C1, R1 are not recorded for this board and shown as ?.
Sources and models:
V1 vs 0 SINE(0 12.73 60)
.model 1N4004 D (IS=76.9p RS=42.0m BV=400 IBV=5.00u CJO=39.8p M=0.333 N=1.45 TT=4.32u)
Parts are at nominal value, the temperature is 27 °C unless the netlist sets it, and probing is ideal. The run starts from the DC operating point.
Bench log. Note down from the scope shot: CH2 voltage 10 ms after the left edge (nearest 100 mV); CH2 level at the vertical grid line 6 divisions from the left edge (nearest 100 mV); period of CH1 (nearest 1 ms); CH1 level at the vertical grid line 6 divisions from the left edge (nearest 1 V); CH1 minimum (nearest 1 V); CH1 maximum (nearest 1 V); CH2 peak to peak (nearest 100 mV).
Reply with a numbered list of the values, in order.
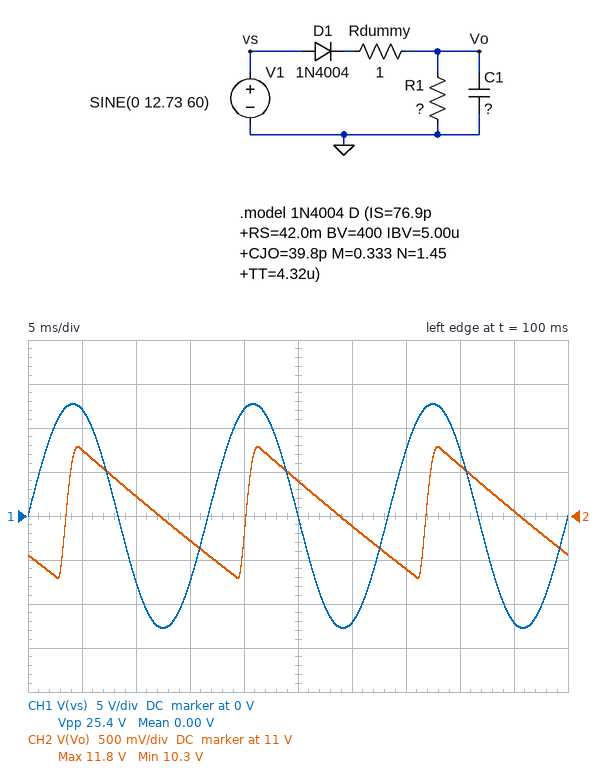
1. 11.2 V
2. 10.9 V
3. 17 ms
4. -12 V
5. -13 V
6. 13 V
7. 1.5 V
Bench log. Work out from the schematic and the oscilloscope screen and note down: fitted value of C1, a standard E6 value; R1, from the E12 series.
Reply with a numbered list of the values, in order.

1. 330 µF
2. 330 Ω
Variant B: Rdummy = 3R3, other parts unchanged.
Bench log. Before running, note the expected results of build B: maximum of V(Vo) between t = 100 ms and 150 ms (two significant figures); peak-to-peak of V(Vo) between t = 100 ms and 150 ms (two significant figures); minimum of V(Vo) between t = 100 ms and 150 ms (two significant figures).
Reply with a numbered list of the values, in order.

1. 11 V
2. 1.4 V
3. 9.9 V
